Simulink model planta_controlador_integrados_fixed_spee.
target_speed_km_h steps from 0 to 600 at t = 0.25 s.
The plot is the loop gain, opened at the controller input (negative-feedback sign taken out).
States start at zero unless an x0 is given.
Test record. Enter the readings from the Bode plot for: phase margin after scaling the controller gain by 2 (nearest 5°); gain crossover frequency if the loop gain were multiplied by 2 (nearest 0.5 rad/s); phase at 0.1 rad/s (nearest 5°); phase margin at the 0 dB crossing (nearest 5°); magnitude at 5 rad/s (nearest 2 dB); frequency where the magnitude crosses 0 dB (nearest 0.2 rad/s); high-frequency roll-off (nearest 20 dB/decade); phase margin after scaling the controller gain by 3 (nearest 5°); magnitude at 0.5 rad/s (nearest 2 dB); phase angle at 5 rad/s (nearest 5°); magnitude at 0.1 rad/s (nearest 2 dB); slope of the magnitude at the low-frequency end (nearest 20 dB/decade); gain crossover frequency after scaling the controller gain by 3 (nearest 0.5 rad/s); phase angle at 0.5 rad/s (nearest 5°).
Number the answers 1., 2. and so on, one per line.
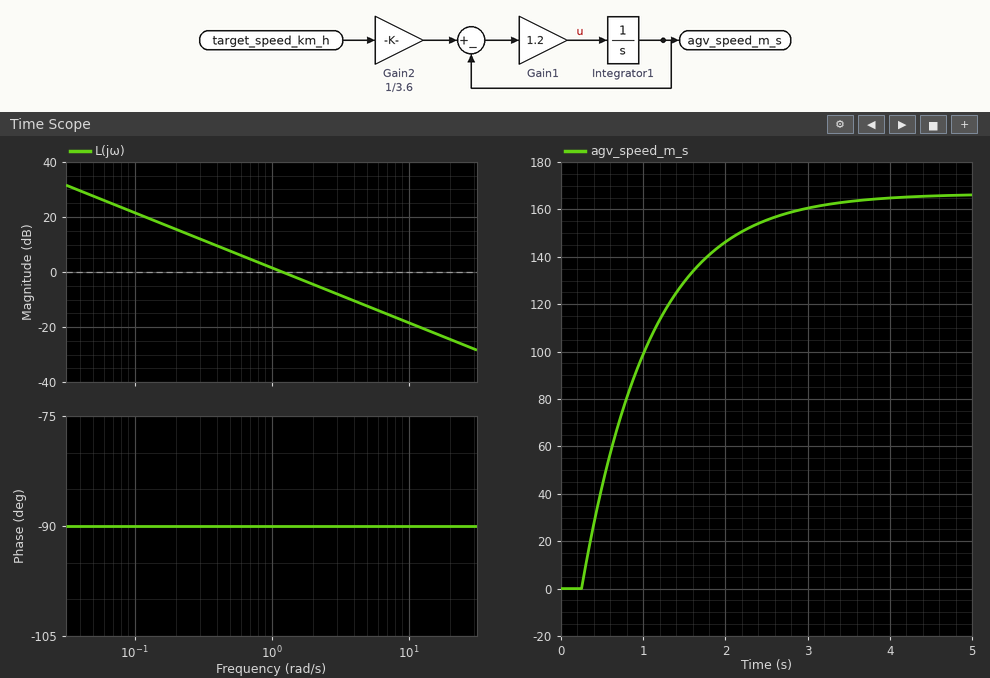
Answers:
1. 90°
2. 2.5 rad/s
3. -90°
4. 90°
5. -12 dB
6. 1.2 rad/s
7. -20 dB/decade
8. 90°
9. 8 dB
10. -90°
11. 22 dB
12. -20 dB/decade
13. 3.5 rad/s
14. -90°
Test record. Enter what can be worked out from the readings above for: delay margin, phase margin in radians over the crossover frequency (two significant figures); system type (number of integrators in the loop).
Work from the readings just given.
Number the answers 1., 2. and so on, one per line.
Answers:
1. 1.3 s
2. 1
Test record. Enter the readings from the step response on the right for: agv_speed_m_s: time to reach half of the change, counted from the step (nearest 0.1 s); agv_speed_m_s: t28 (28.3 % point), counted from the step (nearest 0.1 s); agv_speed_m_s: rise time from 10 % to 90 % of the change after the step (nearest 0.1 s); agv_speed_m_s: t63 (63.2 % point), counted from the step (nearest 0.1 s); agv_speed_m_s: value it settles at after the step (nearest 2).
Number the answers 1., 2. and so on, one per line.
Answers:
1. 0.6 s
2. 0.3 s
3. 1.8 s
4. 0.8 s
5. 166
